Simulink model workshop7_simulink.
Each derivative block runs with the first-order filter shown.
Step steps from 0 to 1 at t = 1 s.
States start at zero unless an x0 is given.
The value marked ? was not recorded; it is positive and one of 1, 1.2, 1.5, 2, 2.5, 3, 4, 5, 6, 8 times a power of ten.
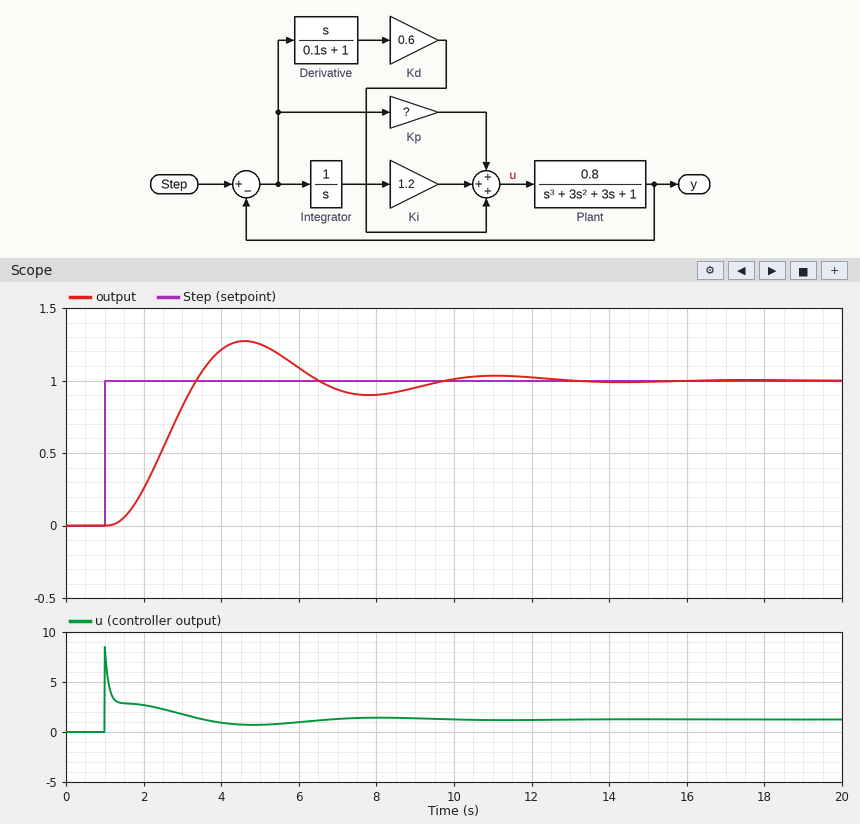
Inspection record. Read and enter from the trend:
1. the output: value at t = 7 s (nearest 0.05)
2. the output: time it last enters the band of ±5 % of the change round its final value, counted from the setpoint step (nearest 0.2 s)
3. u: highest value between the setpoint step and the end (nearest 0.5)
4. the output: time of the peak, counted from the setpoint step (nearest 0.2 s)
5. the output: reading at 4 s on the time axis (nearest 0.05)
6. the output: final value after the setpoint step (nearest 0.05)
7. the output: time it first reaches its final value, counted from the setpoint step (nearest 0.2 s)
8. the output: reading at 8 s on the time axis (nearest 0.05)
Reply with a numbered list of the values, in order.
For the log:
1. 0.95
2. 8.0 s
3. 8.5
4. 3.6 s
5. 1.20
6. 1.00
7. 2.4 s
8. 0.90
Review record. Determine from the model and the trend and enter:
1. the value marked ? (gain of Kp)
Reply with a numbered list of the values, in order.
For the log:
1. 2.5
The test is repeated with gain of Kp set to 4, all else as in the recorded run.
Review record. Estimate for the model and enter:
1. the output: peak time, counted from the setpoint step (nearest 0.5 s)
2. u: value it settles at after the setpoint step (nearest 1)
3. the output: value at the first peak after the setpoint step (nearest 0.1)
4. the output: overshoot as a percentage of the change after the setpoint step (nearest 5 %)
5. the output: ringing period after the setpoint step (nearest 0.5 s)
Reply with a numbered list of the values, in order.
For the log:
1. 3.0 s
2. 1
3. 1.3
4. 35 %
5. 5.0 s
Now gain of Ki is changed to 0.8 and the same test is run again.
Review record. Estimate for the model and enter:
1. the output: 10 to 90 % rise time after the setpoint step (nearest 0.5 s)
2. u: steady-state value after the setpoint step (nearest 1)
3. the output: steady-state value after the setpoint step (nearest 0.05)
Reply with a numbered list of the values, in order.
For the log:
1. 1.5 s
2. 1
3. 1.00
